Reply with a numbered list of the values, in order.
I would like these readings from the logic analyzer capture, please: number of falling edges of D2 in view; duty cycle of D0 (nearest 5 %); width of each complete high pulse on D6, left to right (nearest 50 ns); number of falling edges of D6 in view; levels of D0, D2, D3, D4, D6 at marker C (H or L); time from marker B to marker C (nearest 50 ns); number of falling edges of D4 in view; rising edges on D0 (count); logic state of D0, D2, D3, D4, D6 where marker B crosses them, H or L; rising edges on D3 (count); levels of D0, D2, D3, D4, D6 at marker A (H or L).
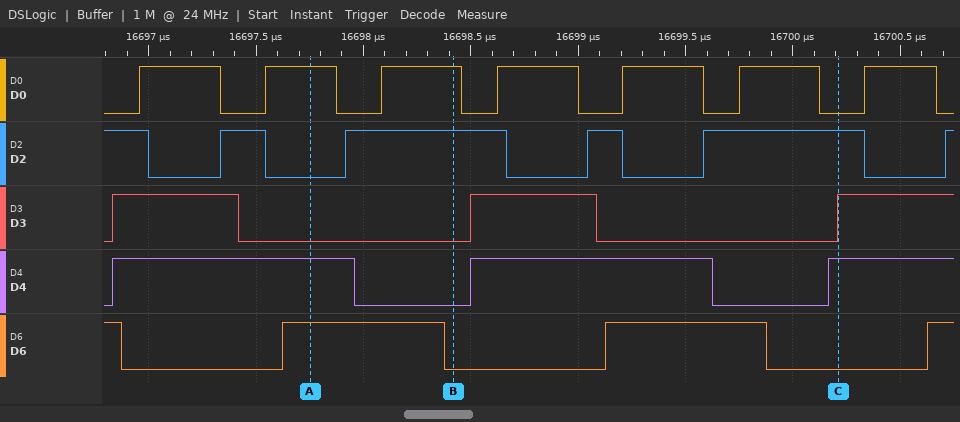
1. 5
2. 65 %
3. 750 ns, 750 ns
4. 3
5. D0=L, D2=H, D3=H, D4=H, D6=L
6. 1800 ns
7. 2
8. 7
9. D0=H, D2=H, D3=L, D4=L, D6=L
10. 3
11. D0=H, D2=L, D3=L, D4=H, D6=H
